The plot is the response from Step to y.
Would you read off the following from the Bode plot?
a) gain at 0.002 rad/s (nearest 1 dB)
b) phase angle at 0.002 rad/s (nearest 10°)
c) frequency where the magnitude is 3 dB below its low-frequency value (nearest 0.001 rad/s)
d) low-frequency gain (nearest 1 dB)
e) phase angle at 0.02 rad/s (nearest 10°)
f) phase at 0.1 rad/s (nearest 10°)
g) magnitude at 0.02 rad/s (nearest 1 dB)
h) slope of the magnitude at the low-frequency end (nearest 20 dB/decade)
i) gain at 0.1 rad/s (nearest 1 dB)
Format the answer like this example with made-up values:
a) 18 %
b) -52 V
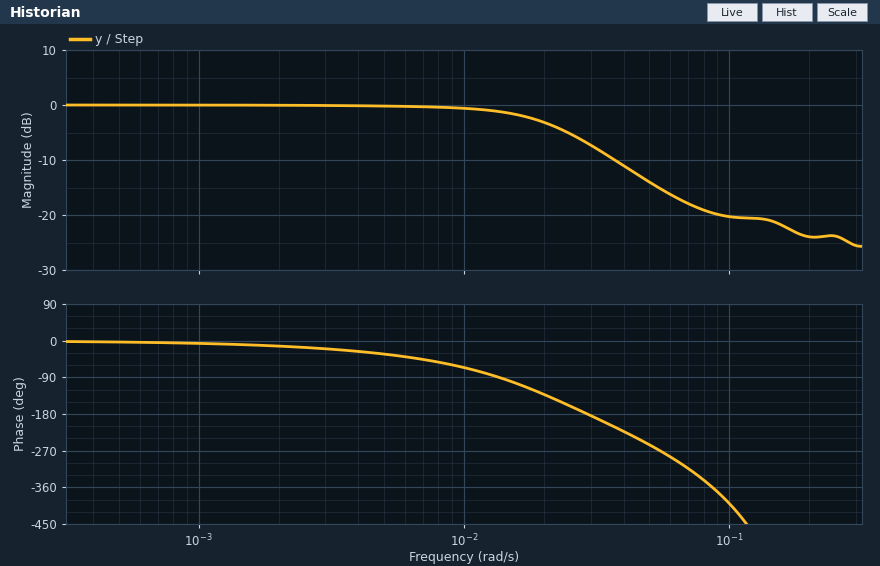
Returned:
a) 0 dB
b) -10°
c) 0.020 rad/s
d) 0 dB
e) -130°
f) -400°
g) -3 dB
h) 0 dB/decade
i) -20 dB
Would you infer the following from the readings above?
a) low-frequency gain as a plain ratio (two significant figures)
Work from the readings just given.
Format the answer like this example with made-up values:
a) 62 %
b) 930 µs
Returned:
a) 1.0
